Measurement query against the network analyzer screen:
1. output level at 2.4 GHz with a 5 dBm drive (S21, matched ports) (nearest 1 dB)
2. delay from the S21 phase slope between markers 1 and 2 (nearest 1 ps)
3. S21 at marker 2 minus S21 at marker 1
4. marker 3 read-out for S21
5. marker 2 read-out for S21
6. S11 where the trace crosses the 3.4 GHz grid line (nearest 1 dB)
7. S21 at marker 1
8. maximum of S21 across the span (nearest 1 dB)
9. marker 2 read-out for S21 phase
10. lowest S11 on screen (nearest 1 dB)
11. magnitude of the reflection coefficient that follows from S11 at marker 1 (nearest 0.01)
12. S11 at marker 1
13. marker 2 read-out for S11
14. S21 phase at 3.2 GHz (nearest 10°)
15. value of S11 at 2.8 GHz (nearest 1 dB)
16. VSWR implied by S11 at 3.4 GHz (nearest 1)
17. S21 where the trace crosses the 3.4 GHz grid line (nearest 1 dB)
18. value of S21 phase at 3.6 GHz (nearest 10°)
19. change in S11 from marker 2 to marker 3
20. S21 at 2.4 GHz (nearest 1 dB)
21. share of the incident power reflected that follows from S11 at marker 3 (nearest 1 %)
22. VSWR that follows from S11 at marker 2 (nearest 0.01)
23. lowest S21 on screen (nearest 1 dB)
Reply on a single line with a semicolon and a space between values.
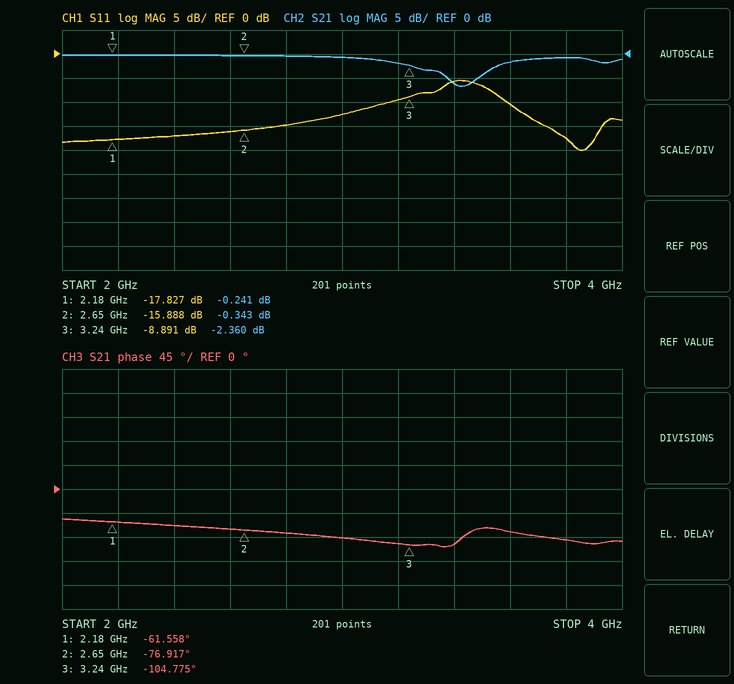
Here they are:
5 dBm; 91 ps; -0.102 dB; -2.360 dB; -0.343 dB; -6 dB; -0.241 dB; 0 dB; -76.917°; -20 dB; 0.13; -17.827 dB; -15.888 dB; -100°; -15 dB; 3; -6 dB; -80°; 6.997 dB; 0 dB; 13 %; 1.38; -7 dB
